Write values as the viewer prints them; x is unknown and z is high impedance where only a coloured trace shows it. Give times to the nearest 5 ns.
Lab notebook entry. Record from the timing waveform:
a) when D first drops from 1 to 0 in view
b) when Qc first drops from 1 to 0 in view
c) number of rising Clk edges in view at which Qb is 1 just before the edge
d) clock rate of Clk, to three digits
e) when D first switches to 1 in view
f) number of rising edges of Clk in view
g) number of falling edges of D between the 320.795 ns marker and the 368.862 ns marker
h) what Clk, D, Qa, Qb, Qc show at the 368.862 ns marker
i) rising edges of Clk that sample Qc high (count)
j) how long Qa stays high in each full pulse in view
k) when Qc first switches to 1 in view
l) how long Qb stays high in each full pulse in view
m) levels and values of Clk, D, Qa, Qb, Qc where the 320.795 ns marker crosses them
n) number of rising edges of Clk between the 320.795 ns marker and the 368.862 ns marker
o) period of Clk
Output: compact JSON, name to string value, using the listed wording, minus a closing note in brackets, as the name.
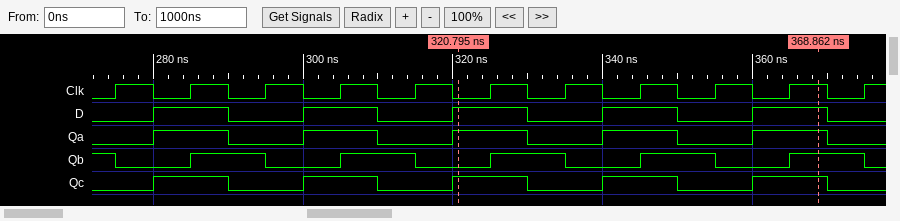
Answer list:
{"when D first drops from 1 to 0 in view": "290 ns", "when Qc first drops from 1 to 0 in view": "290 ns", "number of rising Clk edges in view at which Qb is 1 just before the edge": "6", "clock rate of Clk, to three digits": "100 MHz", "when D first switches to 1 in view": "280 ns", "number of rising edges of Clk in view": "11", "number of falling edges of D between the 320.795 ns marker and the 368.862 ns marker": "2", "what Clk, D, Qa, Qb, Qc show at the 368.862 ns marker": "Clk=1, D=1, Qa=1, Qb=1, Qc=1", "rising edges of Clk that sample Qc high": "5", "how long Qa stays high in each full pulse in view": "10 ns, 10 ns, 10 ns, 10 ns, 10 ns", "when Qc first switches to 1 in view": "280 ns", "how long Qb stays high in each full pulse in view": "10 ns, 10 ns, 10 ns, 10 ns, 10 ns", "levels and values of Clk, D, Qa, Qb, Qc where the 320.795 ns marker crosses them": "Clk=0, D=1, Qa=1, Qb=0, Qc=1", "number of rising edges of Clk between the 320.795 ns marker and the 368.862 ns marker": "5", "period of Clk": "10 ns"}
